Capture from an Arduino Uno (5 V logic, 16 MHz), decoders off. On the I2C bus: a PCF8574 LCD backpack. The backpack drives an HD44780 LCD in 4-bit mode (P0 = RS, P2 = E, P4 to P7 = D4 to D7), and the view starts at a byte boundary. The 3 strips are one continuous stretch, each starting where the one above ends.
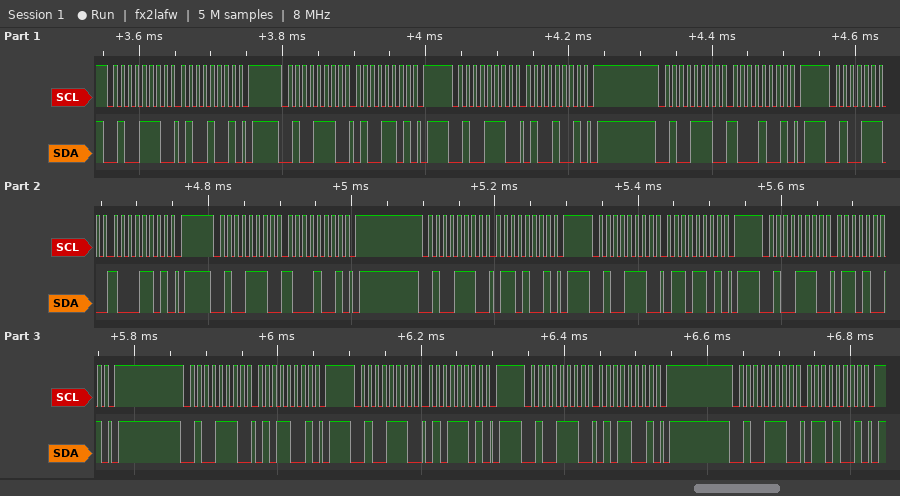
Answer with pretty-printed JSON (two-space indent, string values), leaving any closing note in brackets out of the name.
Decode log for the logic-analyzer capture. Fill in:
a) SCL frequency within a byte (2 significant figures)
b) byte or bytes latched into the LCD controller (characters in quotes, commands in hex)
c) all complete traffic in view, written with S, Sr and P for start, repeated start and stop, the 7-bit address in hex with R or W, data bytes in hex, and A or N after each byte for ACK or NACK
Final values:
{
  "SCL frequency within a byte": "100 kHz",
  "byte or bytes latched into the LCD controller": "'H' 'e'",
  "all complete traffic in view, written with S, Sr and P for start, repeated start and stop, the 7-bit address in hex with R or W, data bytes in hex, and A or N after each byte for ACK or NACK": "S 27W A 49 A P S 27W A 4D A P S 27W A 49 A P S 27W A 89 A P S 27W A 8D A P S 27W A 89 A P S 27W A 69 A P S 27W A 6D A P S 27W A 69 A P S 27W A 59 A P S 27W A 5D A P S 27W A 59 A P S 27W A 69 A P"
}
